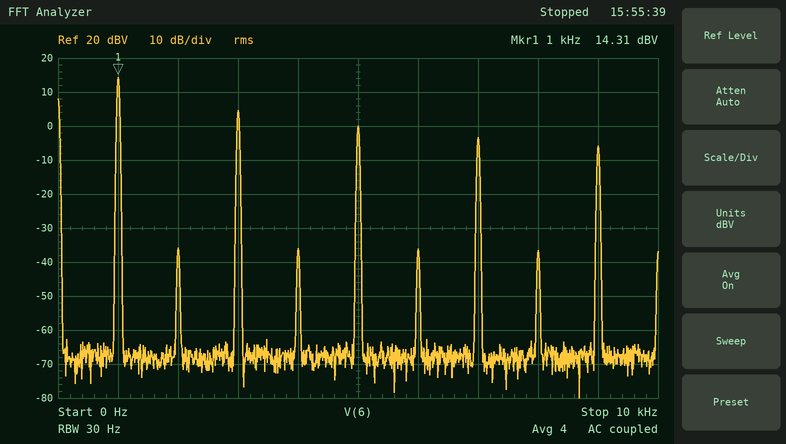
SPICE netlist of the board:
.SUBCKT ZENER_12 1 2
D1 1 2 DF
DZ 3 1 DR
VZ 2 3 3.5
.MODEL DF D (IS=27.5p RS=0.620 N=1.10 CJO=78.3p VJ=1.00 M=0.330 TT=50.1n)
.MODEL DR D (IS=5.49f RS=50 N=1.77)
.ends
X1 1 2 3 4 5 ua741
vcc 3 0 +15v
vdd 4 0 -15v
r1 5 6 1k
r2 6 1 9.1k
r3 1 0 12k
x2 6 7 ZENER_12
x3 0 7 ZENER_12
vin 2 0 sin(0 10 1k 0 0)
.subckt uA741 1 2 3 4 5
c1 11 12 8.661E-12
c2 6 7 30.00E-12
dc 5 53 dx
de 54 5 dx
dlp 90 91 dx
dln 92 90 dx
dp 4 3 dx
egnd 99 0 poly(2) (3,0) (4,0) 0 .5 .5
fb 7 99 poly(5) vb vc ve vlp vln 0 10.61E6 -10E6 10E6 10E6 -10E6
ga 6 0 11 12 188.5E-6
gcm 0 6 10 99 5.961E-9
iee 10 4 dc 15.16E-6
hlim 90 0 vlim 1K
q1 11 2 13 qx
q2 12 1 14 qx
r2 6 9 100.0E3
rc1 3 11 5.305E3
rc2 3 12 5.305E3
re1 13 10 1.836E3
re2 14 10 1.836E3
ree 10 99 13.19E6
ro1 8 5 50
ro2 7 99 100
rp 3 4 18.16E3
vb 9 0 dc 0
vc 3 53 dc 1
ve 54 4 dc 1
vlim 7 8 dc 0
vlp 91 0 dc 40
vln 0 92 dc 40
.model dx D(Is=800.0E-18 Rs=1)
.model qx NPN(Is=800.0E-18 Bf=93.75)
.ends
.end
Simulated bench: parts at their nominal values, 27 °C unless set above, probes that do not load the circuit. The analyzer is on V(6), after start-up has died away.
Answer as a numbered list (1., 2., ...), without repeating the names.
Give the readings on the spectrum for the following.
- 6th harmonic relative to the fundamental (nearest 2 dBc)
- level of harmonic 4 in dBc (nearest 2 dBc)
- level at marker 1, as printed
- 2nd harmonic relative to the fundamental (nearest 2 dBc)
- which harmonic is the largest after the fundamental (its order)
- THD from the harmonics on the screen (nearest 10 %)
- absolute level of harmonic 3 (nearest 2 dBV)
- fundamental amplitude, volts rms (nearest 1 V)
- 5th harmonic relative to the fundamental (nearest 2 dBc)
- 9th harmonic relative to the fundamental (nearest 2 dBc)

1. -50 dBc
2. -50 dBc
3. 14.31 dBV
4. -50 dBc
5. 3
6. 40 %
7. 4 dBV
8. 5 V
9. -14 dBc
10. -20 dBc
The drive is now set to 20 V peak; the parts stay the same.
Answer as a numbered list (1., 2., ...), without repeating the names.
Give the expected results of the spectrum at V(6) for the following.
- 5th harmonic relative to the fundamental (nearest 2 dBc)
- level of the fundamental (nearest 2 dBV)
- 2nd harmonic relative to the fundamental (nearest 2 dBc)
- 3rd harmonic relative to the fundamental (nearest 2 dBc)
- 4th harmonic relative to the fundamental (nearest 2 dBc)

1. -4 dBc
2. 6 dBV
3. 2 dBc
4. 4 dBc
5. -20 dBc
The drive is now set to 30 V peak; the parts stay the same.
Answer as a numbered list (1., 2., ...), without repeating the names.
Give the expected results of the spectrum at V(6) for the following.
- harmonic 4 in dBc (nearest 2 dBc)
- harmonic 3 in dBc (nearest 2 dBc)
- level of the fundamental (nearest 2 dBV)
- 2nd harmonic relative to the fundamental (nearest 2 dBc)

1. 2 dBc
2. 2 dBc
3. 0 dBV
4. 6 dBc
